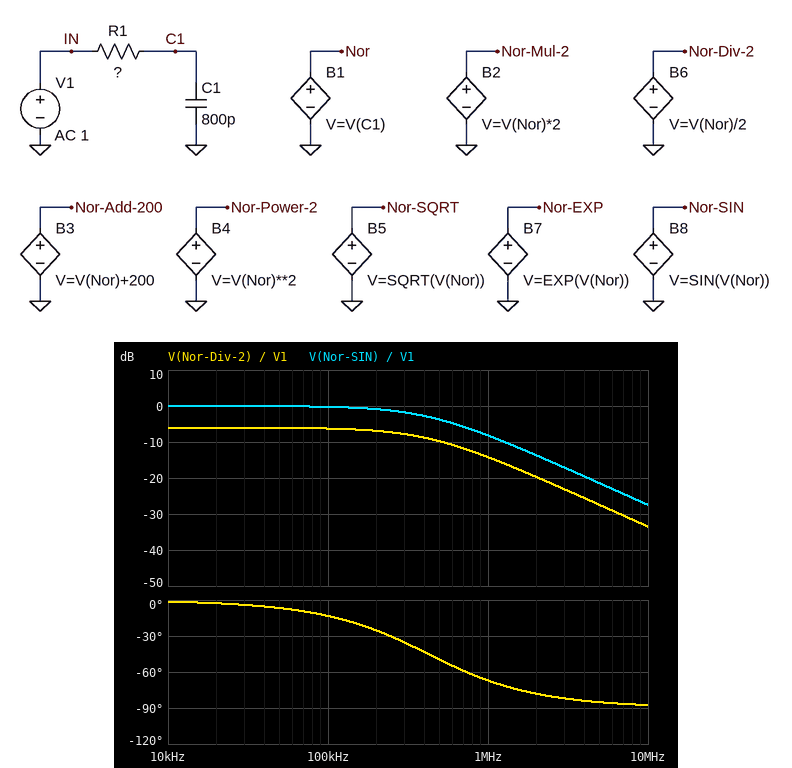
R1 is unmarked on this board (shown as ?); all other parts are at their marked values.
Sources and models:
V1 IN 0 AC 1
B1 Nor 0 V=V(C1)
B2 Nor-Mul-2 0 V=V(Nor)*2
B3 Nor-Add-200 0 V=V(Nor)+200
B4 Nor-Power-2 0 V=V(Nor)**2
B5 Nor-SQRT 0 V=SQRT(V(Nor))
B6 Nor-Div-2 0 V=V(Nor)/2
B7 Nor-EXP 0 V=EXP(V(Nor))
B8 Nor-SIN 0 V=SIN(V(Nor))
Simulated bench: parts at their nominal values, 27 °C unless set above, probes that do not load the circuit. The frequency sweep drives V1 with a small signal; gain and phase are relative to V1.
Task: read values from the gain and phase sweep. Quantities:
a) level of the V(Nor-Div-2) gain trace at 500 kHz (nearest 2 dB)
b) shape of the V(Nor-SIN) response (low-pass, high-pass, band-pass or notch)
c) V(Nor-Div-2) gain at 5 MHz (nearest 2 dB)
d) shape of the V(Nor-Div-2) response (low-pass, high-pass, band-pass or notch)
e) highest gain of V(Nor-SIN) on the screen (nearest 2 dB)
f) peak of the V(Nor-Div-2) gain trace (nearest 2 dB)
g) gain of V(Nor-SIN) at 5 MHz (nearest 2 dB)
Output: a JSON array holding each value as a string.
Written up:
["-10 dB", "low-pass", "-28 dB", "low-pass", "0 dB", "-6 dB", "-22 dB"]
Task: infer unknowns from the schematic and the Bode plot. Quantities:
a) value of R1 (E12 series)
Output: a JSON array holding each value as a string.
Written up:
["470 Ω"]
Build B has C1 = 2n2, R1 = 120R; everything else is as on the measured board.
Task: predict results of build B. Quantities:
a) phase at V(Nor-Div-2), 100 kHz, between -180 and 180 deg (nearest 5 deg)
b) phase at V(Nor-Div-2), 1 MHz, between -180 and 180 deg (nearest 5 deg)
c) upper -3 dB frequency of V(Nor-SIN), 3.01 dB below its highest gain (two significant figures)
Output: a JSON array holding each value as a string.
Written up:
["-10 deg", "-60 deg", "600 kHz"]
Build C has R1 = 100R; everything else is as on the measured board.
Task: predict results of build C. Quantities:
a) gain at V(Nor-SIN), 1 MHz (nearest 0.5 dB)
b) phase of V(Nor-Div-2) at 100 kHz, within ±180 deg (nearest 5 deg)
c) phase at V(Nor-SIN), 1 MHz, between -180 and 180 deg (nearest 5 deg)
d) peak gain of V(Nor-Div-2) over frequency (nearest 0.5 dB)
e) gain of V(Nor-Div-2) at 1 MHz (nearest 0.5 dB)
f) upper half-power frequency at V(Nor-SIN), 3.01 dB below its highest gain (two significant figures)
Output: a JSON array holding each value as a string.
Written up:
["-1.0 dB", "-5 deg", "-25 deg", "-6.0 dB", "-7.0 dB", "2.0 MHz"]
